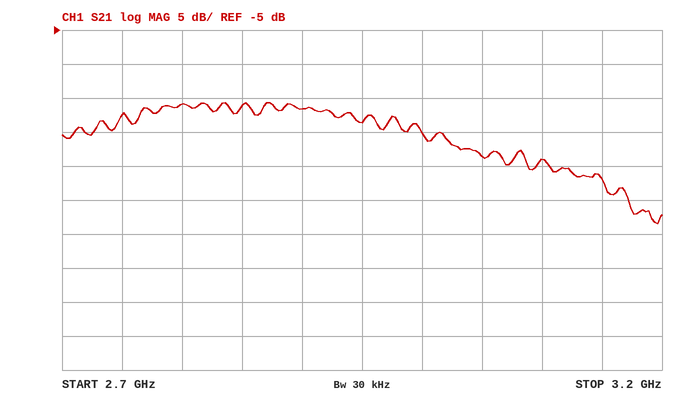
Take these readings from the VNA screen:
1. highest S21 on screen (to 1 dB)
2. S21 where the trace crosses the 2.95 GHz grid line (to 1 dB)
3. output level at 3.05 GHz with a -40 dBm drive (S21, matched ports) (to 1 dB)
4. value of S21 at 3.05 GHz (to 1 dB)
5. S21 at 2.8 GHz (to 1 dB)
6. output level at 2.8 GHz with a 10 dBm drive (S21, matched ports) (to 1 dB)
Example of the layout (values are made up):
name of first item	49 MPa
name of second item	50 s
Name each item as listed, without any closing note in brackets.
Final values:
highest S21 on screen	-16 dB
S21 where the trace crosses the 2.95 GHz grid line	-19 dB
output level at 3.05 GHz with a -40 dBm drive (S21, matched ports)	-64 dBm
value of S21 at 3.05 GHz	-24 dB
S21 at 2.8 GHz	-16 dB
output level at 2.8 GHz with a 10 dBm drive (S21, matched ports)	-6 dBm
